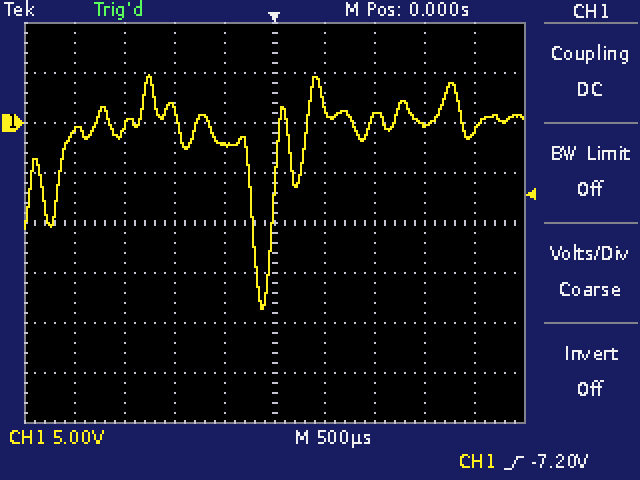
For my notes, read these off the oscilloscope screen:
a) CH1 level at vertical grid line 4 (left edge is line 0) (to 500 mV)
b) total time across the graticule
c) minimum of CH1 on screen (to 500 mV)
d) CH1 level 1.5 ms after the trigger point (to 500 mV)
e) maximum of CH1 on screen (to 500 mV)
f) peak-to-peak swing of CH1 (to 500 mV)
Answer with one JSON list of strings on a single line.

["-2.0 V", "5 ms", "-18.5 V", "0.0 V", "5.0 V", "23.5 V"]
